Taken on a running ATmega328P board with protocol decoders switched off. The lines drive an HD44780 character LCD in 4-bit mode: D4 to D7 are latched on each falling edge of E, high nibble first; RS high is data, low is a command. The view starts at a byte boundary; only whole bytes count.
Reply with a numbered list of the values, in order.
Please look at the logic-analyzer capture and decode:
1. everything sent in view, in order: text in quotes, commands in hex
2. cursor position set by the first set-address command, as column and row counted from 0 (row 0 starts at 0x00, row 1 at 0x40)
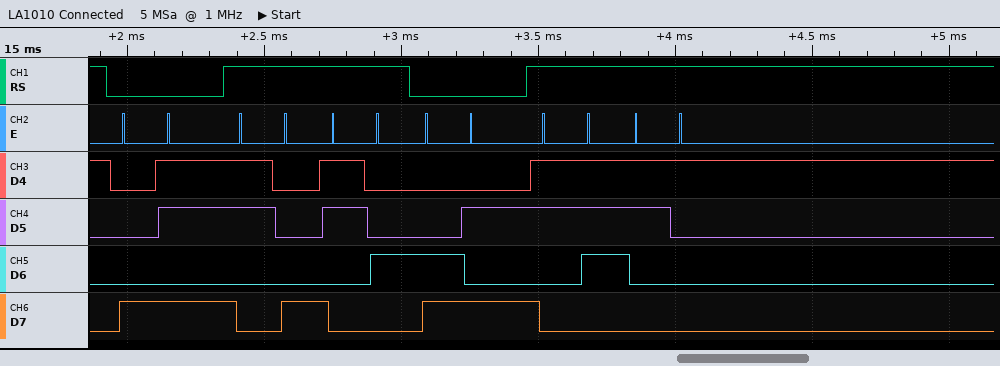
1. 0x8B "84" 0xCA "71"
2. column 11, row 0
